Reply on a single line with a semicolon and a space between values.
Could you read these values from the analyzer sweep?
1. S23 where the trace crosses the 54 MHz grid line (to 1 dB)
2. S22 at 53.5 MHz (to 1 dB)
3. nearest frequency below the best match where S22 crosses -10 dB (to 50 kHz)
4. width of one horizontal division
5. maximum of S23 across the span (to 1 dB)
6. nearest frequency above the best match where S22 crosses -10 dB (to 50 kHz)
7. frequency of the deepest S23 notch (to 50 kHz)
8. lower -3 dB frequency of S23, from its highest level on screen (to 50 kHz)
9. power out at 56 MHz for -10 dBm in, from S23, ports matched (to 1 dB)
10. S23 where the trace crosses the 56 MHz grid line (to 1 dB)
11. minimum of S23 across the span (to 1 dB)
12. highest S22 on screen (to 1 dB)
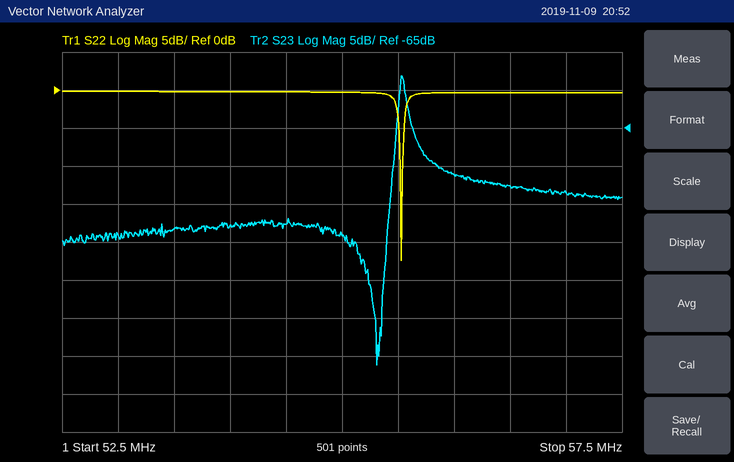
-78 dB; 0 dB; 55.50 MHz; 500 kHz; -58 dB; 55.55 MHz; 55.30 MHz; 55.50 MHz; -81 dBm; -71 dB; -96 dB; 0 dB
